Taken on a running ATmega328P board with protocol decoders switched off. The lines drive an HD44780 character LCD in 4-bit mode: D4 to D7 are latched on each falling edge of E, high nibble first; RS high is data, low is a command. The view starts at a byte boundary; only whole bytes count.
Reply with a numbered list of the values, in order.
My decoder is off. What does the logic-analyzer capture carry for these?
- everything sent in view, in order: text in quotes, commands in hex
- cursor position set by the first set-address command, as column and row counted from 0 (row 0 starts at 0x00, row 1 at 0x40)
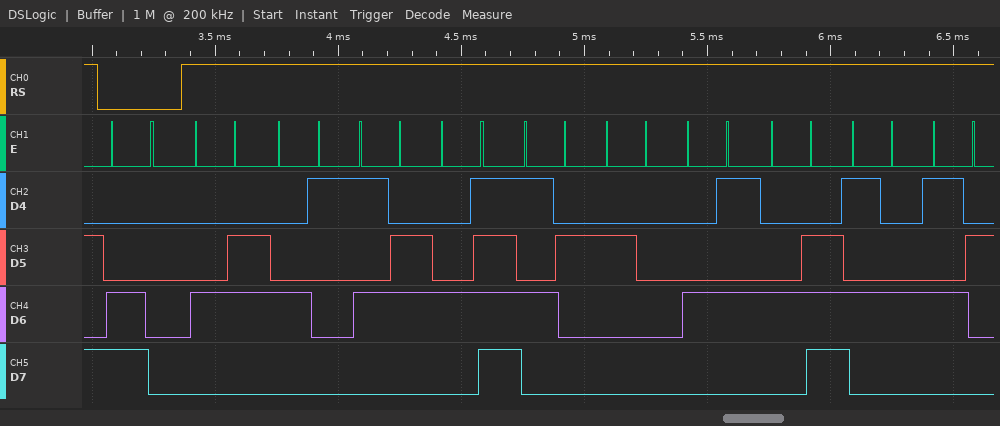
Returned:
1. 0xC0 "FAVOR ENTR"
2. column 0, row 1
